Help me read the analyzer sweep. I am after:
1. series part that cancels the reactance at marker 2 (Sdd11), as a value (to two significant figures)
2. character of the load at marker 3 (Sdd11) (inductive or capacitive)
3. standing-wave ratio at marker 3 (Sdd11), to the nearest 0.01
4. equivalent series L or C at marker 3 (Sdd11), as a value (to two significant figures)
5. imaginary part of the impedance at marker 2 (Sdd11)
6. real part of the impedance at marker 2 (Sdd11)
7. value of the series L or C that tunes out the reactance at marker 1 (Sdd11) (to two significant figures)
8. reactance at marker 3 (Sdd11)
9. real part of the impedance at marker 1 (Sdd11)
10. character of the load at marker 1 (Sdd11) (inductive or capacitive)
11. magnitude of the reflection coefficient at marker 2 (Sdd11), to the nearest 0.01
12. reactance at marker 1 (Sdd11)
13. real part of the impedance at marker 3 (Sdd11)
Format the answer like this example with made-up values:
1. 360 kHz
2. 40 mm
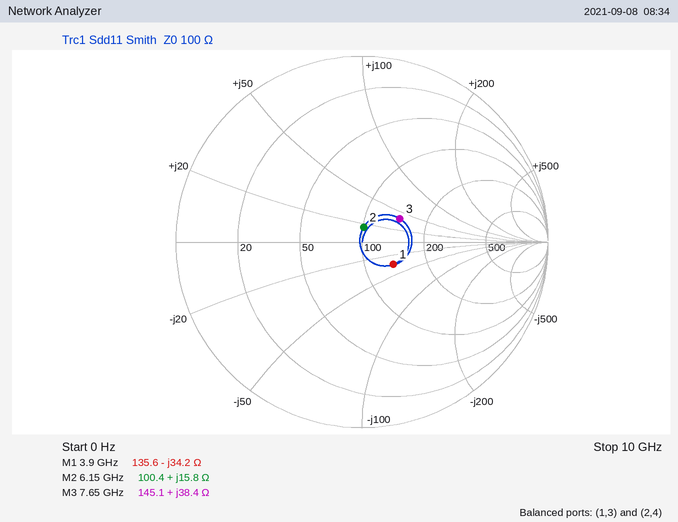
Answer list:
1. 1.6 pF
2. inductive
3. 1.63
4. 800 pH
5. +15.8 Ω
6. 100.4 Ω
7. 1.4 nH
8. +38.4 Ω
9. 135.6 Ω
10. capacitive
11. 0.08
12. -34.2 Ω
13. 145.1 Ω
